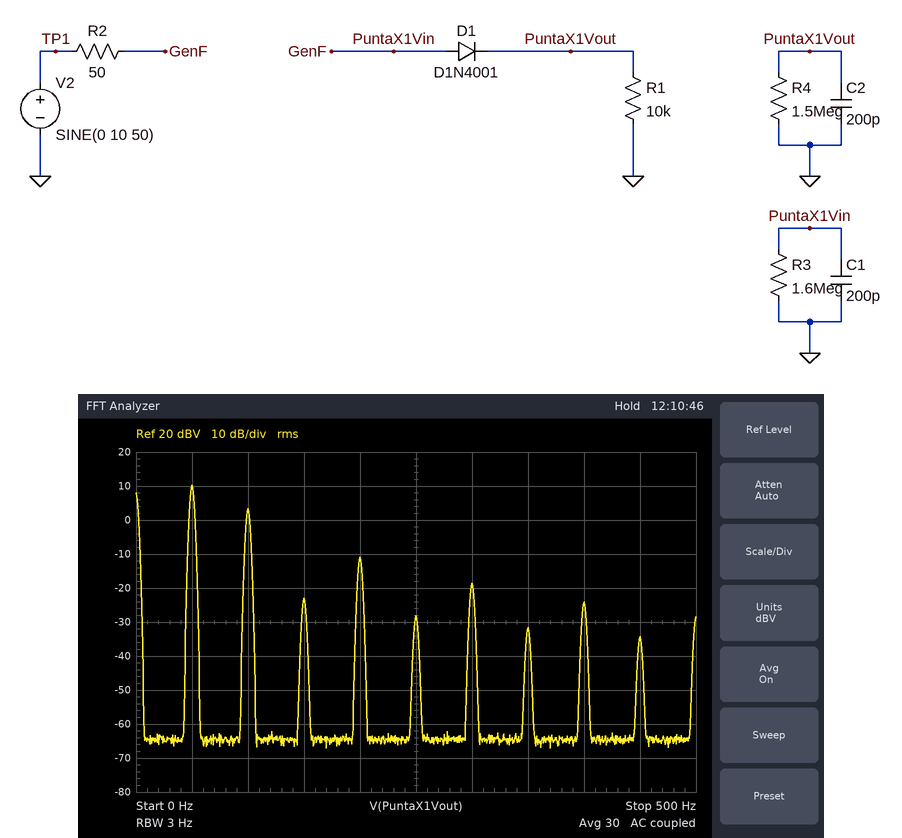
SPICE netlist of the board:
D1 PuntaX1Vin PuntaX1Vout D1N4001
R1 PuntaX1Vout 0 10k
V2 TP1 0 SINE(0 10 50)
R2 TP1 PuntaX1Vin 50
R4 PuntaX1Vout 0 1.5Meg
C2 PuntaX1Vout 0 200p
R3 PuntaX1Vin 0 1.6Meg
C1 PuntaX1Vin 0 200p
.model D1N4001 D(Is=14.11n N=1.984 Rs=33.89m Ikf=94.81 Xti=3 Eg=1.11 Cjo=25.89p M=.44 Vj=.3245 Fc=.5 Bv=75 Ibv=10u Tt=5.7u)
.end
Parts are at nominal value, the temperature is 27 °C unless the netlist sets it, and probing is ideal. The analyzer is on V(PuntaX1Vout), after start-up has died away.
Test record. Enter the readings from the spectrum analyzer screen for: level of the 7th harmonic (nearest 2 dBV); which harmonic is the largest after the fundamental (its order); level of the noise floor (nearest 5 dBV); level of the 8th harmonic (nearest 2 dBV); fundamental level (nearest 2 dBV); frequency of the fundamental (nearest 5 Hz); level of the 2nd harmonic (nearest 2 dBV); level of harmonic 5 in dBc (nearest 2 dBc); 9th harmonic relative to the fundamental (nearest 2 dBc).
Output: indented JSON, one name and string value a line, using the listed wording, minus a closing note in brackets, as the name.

{
  "level of the 7th harmonic": "-32 dBV",
  "which harmonic is the largest after the fundamental": "2",
  "level of the noise floor": "-65 dBV",
  "level of the 8th harmonic": "-24 dBV",
  "fundamental level": "10 dBV",
  "frequency of the fundamental": "50 Hz",
  "level of the 2nd harmonic": "4 dBV",
  "level of harmonic 5 in dBc": "-38 dBc",
  "9th harmonic relative to the fundamental": "-44 dBc"
}
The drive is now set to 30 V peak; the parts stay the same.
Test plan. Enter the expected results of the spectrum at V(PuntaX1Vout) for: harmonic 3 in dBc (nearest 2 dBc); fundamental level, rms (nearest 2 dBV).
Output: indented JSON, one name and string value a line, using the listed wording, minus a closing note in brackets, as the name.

{
  "harmonic 3 in dBc": "-42 dBc",
  "fundamental level, rms": "20 dBV"
}
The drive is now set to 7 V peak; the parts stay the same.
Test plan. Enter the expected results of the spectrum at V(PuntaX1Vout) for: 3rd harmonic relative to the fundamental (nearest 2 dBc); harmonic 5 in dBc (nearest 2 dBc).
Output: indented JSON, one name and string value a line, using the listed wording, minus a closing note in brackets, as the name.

{
  "3rd harmonic relative to the fundamental": "-30 dBc",
  "harmonic 5 in dBc": "-36 dBc"
}
